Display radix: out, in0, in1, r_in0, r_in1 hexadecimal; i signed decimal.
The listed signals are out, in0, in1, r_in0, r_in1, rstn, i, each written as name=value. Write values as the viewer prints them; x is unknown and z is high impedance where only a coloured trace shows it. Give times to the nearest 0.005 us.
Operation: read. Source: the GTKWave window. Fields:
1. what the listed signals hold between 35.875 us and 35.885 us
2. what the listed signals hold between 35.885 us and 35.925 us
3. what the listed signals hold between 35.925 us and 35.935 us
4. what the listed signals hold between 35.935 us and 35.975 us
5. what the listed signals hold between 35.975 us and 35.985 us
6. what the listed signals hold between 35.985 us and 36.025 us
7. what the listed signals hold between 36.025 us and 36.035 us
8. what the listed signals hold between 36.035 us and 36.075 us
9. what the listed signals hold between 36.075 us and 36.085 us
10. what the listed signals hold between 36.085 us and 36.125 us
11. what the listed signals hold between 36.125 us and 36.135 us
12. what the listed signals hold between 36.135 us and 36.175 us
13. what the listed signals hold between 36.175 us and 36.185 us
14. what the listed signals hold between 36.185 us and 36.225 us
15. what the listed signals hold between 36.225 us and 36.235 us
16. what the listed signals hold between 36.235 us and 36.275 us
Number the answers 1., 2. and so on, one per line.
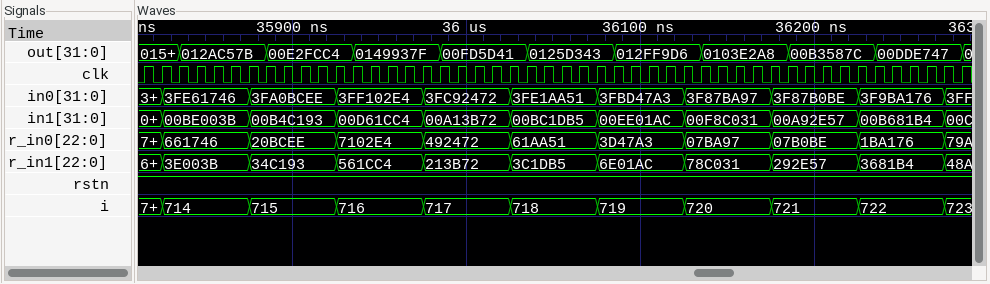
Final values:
1. out=012AC57B, in0=3FA0BCEE, in1=00B4C193, r_in0=20BCEE, r_in1=34C193, rstn=1, i=715
2. out=00E2FCC4, in0=3FA0BCEE, in1=00B4C193, r_in0=20BCEE, r_in1=34C193, rstn=1, i=715
3. out=00E2FCC4, in0=3FF102E4, in1=00D61CC4, r_in0=7102E4, r_in1=561CC4, rstn=1, i=716
4. out=0149937F, in0=3FF102E4, in1=00D61CC4, r_in0=7102E4, r_in1=561CC4, rstn=1, i=716
5. out=0149937F, in0=3FC92472, in1=00A13B72, r_in0=492472, r_in1=213B72, rstn=1, i=717
6. out=00FD5D41, in0=3FC92472, in1=00A13B72, r_in0=492472, r_in1=213B72, rstn=1, i=717
7. out=00FD5D41, in0=3FE1AA51, in1=00BC1DB5, r_in0=61AA51, r_in1=3C1DB5, rstn=1, i=718
8. out=0125D343, in0=3FE1AA51, in1=00BC1DB5, r_in0=61AA51, r_in1=3C1DB5, rstn=1, i=718
9. out=0125D343, in0=3FBD47A3, in1=00EE01AC, r_in0=3D47A3, r_in1=6E01AC, rstn=1, i=719
10. out=012FF9D6, in0=3FBD47A3, in1=00EE01AC, r_in0=3D47A3, r_in1=6E01AC, rstn=1, i=719
11. out=012FF9D6, in0=3F87BA97, in1=00F8C031, r_in0=07BA97, r_in1=78C031, rstn=1, i=720
12. out=0103E2A8, in0=3F87BA97, in1=00F8C031, r_in0=07BA97, r_in1=78C031, rstn=1, i=720
13. out=0103E2A8, in0=3F87B0BE, in1=00A92E57, r_in0=07B0BE, r_in1=292E57, rstn=1, i=721
14. out=00B3587C, in0=3F87B0BE, in1=00A92E57, r_in0=07B0BE, r_in1=292E57, rstn=1, i=721
15. out=00B3587C, in0=3F9BA176, in1=00B681B4, r_in0=1BA176, r_in1=3681B4, rstn=1, i=722
16. out=00DDE747, in0=3F9BA176, in1=00B681B4, r_in0=1BA176, r_in1=3681B4, rstn=1, i=722
